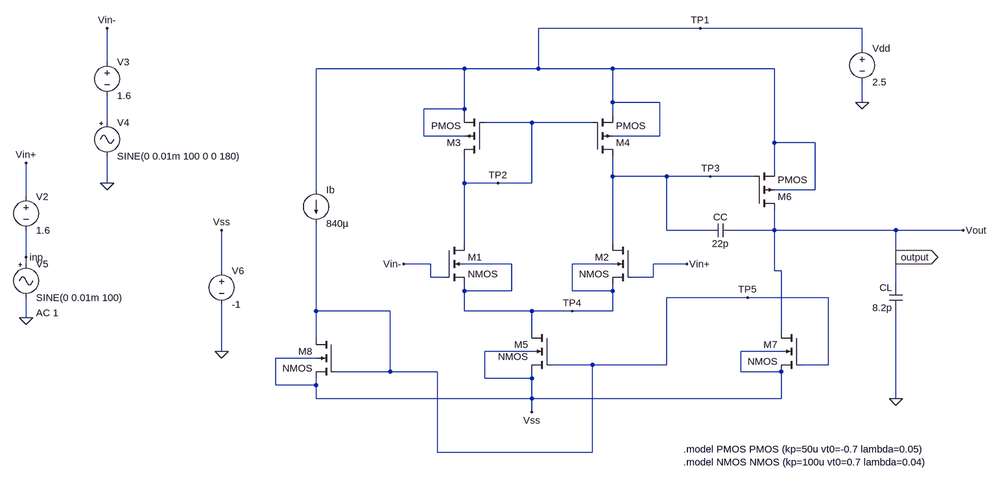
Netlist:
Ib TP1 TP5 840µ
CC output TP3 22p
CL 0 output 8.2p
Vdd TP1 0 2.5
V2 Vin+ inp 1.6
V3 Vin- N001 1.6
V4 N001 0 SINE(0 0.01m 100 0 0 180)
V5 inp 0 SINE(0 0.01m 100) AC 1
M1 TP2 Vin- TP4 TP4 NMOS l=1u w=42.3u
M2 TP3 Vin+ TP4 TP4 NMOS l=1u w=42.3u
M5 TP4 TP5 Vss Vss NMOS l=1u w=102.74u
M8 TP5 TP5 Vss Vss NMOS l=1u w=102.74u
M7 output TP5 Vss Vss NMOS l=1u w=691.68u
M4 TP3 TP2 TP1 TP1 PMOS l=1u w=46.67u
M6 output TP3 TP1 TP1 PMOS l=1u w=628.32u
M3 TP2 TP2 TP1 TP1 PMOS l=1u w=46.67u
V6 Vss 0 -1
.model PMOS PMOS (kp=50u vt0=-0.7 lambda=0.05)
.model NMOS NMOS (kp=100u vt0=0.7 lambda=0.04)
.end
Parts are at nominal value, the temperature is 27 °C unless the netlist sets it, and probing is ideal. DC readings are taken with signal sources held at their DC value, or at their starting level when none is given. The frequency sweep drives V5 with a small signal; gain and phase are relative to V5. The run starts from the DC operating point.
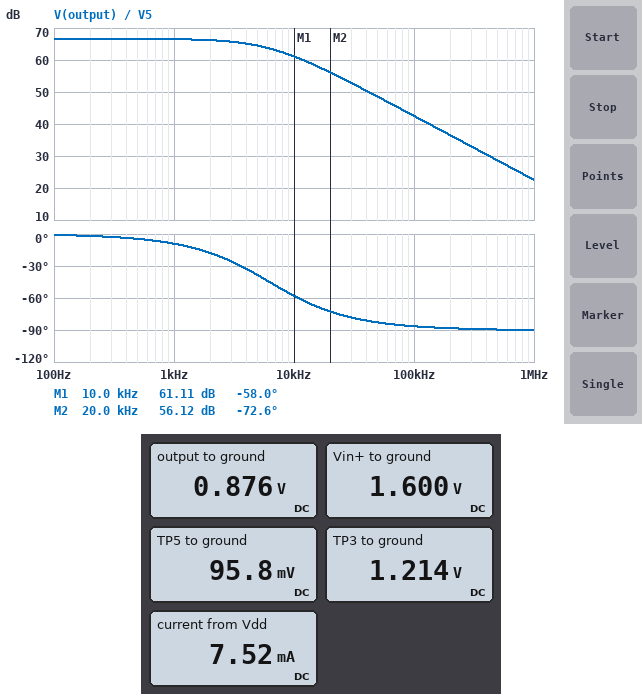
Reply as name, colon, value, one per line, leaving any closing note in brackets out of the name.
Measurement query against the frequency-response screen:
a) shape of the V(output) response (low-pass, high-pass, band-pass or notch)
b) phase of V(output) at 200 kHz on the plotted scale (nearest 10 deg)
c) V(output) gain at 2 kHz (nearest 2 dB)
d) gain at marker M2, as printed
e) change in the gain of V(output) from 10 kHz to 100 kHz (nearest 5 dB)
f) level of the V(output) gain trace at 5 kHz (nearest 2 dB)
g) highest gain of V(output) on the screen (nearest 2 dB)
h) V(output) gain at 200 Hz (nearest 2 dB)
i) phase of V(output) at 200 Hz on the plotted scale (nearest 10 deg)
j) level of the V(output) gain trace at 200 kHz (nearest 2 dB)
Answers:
shape of the V(output) response: low-pass
phase of V(output) at 200 kHz on the plotted scale: -90 deg
V(output) gain at 2 kHz: 66 dB
gain at marker M2, as printed: 56.12 dB
change in the gain of V(output) from 10 kHz to 100 kHz: -20 dB
level of the V(output) gain trace at 5 kHz: 64 dB
highest gain of V(output) on the screen: 66 dB
V(output) gain at 200 Hz: 66 dB
phase of V(output) at 200 Hz on the plotted scale: 0 deg
level of the V(output) gain trace at 200 kHz: 36 dB
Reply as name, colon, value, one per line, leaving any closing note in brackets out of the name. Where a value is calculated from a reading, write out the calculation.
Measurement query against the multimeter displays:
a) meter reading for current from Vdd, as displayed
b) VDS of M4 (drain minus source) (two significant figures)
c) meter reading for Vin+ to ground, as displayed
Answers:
meter reading for current from Vdd, as displayed: 7.52 mA
VDS of M4 (drain minus source): 1.214 V - 2.5 V = -1.3 V
meter reading for Vin+ to ground, as displayed: 1.600 V
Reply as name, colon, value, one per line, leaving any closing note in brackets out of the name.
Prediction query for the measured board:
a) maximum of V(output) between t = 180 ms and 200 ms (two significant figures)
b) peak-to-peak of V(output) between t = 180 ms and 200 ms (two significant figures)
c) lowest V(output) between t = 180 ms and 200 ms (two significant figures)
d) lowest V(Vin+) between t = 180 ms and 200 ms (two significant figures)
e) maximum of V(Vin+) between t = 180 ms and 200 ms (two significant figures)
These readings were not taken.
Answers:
maximum of V(output) between t = 180 ms and 200 ms: 920 mV
peak-to-peak of V(output) between t = 180 ms and 200 ms: 86 mV
lowest V(output) between t = 180 ms and 200 ms: 830 mV
lowest V(Vin+) between t = 180 ms and 200 ms: 1.6 V
maximum of V(Vin+) between t = 180 ms and 200 ms: 1.6 V
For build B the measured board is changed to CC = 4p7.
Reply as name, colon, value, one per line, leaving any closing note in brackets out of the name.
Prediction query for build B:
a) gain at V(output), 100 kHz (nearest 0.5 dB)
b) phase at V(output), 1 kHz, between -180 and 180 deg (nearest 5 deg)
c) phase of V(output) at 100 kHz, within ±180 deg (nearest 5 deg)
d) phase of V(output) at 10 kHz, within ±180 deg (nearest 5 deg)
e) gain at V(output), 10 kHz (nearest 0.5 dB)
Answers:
gain at V(output), 100 kHz: 55.5 dB
phase at V(output), 1 kHz, between -180 and 180 deg: 0 deg
phase of V(output) at 100 kHz, within ±180 deg: -75 deg
phase of V(output) at 10 kHz, within ±180 deg: -20 deg
gain at V(output), 10 kHz: 66.0 dB
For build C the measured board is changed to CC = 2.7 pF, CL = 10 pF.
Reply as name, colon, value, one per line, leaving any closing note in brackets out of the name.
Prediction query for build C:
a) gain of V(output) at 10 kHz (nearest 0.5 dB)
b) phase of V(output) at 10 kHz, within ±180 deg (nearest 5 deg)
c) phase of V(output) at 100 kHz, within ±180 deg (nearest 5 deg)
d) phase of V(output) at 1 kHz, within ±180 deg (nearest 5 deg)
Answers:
gain of V(output) at 10 kHz: 66.5 dB
phase of V(output) at 10 kHz, within ±180 deg: -10 deg
phase of V(output) at 100 kHz, within ±180 deg: -65 deg
phase of V(output) at 1 kHz, within ±180 deg: 0 deg
